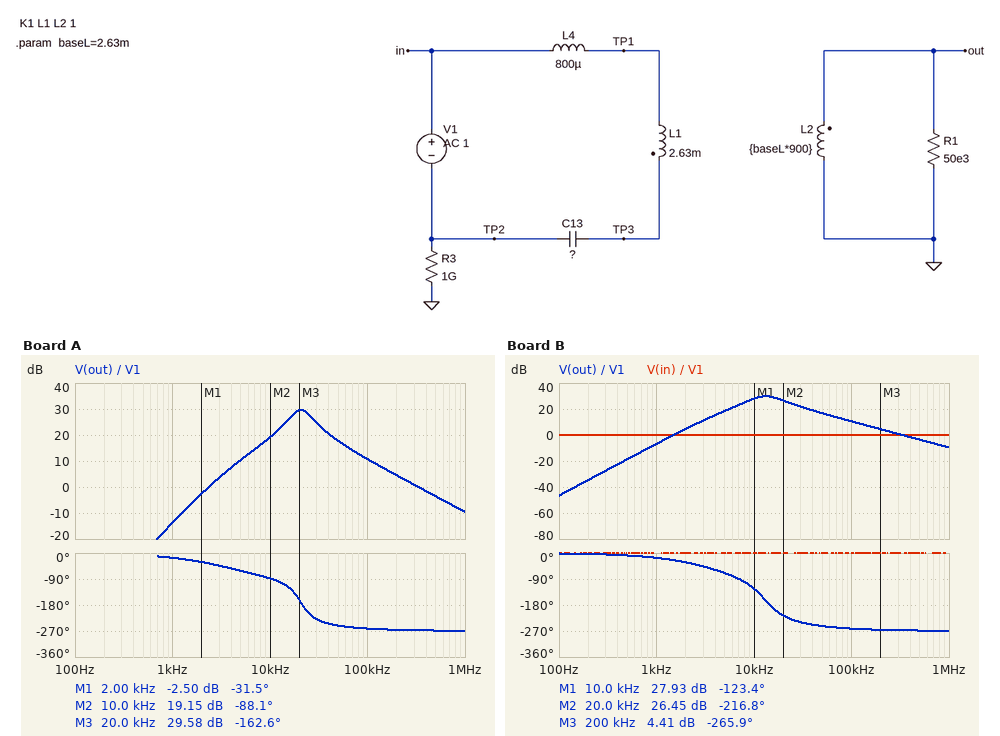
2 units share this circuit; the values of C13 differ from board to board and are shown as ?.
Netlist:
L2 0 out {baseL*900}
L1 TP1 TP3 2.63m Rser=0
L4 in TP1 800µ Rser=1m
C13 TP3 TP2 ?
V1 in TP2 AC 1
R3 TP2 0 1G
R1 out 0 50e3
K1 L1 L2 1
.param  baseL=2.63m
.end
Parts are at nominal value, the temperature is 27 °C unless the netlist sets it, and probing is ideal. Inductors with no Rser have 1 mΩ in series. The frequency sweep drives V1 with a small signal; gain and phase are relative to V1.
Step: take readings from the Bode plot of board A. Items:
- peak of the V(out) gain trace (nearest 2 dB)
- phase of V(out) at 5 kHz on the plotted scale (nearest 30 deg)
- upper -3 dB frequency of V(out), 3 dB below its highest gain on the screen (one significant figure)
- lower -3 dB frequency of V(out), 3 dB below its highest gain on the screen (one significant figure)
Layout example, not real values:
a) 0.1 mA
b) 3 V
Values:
a) 30 dB
b) -60 deg
c) 30 kHz
d) 20 kHz
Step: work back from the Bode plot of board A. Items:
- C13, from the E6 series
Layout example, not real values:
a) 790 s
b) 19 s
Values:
a) 68 nF
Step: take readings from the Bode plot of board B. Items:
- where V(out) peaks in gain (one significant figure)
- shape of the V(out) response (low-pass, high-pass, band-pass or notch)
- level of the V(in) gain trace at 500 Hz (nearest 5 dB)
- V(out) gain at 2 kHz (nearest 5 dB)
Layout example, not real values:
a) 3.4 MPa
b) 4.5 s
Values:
a) 10 kHz
b) band-pass
c) 0 dB
d) 5 dB
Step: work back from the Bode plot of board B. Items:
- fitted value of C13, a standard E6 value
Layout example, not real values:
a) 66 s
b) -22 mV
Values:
a) 150 nF
